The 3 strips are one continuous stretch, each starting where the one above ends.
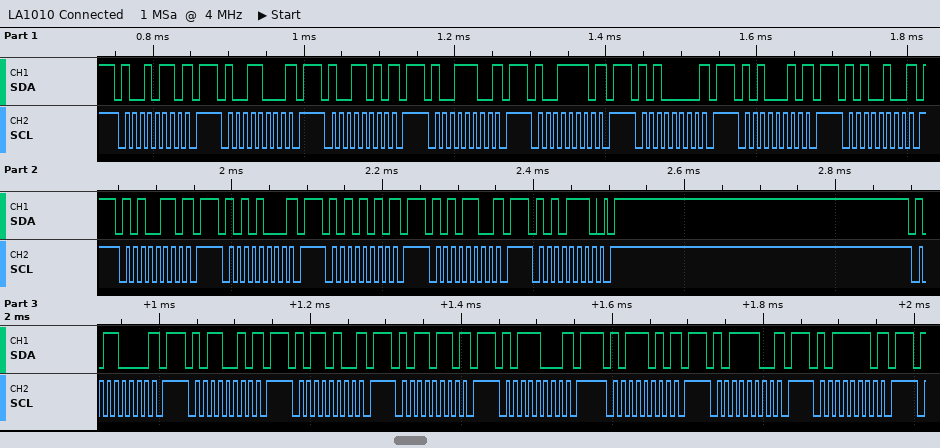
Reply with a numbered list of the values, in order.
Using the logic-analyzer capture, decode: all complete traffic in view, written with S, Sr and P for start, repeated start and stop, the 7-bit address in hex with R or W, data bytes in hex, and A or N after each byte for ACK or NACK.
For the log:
1. S 4BW N P S 4CW N P S 4DW N P S 4EW N P S 4FW N P S 50W N P S 51W N P S 52W N P S 53W N P S 54W N P S 55W N P S 56W N P S 57W A P S 58W N P S 59W N P S 5AW N P S 5BW N P S 5CW N P S 5DW N P S 5EW N P S 5FW N P
